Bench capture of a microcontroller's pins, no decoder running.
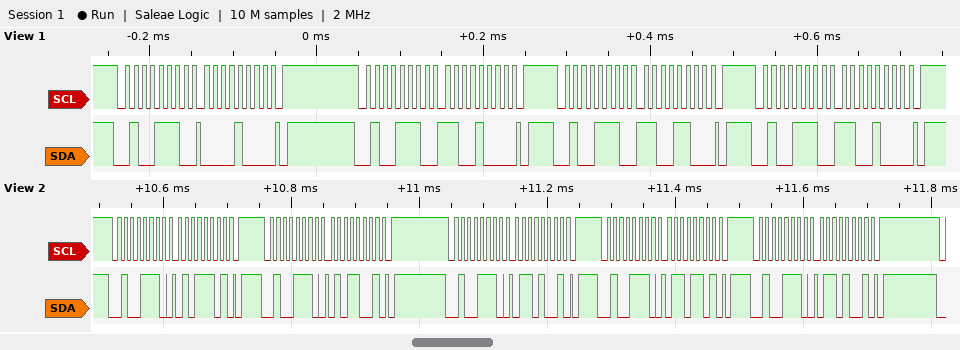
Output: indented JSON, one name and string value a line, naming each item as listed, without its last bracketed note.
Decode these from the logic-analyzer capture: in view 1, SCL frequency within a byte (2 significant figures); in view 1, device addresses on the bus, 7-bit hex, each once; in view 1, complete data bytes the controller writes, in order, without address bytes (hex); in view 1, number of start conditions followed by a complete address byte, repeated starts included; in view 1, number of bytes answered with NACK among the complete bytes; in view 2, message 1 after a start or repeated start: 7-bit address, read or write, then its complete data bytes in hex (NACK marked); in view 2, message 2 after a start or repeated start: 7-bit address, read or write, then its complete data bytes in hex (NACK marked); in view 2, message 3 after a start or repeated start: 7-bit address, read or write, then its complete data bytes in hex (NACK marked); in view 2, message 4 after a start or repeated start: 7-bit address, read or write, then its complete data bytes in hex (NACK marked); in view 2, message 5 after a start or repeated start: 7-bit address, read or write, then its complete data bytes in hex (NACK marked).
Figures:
{
  "in view 1, SCL frequency within a byte": "100 kHz",
  "in view 1, device addresses on the bus, 7-bit hex, each once": "0x27",
  "in view 1, complete data bytes the controller writes, in order, without address bytes": "08 C8 CC C8",
  "in view 1, number of start conditions followed by a complete address byte, repeated starts included": "4",
  "in view 1, number of bytes answered with NACK among the complete bytes": "0",
  "in view 2, message 1 after a start or repeated start: 7-bit address, read or write, then its complete data bytes in hex": "0x27 write: 5D",
  "in view 2, message 2 after a start or repeated start: 7-bit address, read or write, then its complete data bytes in hex": "0x27 write: 59",
  "in view 2, message 3 after a start or repeated start: 7-bit address, read or write, then its complete data bytes in hex": "0x27 write: 69",
  "in view 2, message 4 after a start or repeated start: 7-bit address, read or write, then its complete data bytes in hex": "0x27 write: 6D",
  "in view 2, message 5 after a start or repeated start: 7-bit address, read or write, then its complete data bytes in hex": "0x27 write: 69"
}
